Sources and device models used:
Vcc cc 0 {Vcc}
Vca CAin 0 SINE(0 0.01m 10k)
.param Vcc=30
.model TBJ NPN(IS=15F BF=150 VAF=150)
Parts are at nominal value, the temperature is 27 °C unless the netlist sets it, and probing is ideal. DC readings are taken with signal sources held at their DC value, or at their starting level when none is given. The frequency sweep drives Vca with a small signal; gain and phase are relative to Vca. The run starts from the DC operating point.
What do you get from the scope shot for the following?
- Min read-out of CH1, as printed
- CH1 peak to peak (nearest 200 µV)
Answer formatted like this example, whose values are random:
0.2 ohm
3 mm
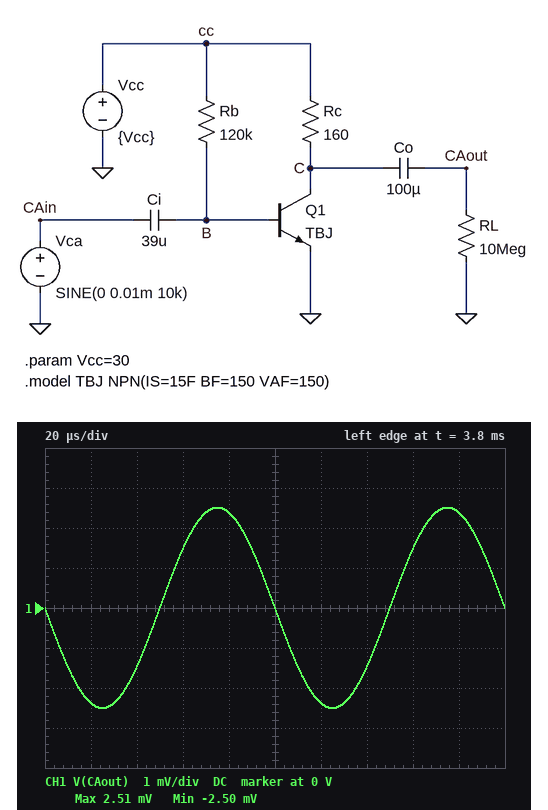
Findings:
-2.50 mV
5.0 mV
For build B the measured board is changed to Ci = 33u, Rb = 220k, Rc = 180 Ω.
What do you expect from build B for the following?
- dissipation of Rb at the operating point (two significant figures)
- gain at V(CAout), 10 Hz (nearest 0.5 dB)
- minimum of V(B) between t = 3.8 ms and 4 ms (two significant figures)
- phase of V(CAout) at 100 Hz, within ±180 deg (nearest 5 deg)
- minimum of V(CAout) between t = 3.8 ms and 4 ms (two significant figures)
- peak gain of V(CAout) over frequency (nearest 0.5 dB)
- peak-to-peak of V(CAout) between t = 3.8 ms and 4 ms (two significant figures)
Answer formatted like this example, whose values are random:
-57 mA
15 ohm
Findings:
3.9 mW
35.5 dB
720 mV
-165 deg
-1.6 mV
44.0 dB
3.2 mV
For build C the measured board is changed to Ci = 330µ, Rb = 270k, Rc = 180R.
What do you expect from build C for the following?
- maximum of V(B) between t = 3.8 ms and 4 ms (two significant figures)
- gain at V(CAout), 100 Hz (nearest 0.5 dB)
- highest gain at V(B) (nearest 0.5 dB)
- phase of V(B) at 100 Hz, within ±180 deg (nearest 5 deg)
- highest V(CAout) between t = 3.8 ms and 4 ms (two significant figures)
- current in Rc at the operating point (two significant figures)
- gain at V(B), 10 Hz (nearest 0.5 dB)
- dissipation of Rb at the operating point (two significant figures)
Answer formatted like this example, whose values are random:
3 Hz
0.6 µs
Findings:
720 mV
42.5 dB
0 dB
0 deg
1.3 mV
19 mA
0 dB
3.2 mW
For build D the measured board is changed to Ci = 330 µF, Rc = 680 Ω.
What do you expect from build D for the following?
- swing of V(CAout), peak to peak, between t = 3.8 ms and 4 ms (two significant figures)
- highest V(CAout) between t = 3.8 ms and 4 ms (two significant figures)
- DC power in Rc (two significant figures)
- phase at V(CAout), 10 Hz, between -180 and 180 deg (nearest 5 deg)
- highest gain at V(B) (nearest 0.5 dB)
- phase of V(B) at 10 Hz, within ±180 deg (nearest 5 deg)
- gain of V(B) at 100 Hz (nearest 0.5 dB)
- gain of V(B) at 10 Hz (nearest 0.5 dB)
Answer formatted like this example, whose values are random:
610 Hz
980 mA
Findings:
17 mV
8.5 mV
960 mW
-155 deg
0 dB
25 deg
0 dB
-1.0 dB
